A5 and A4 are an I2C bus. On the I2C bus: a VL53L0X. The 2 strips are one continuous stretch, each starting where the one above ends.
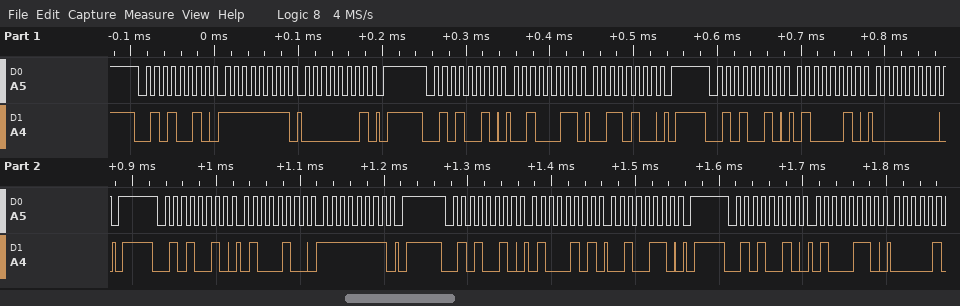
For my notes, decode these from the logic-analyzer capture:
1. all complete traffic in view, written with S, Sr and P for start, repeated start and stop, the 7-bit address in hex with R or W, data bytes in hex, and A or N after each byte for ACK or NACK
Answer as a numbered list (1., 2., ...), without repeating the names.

1. S 29W A FF A 01 A P S 29W A 23 A 34 A P S 29W A 42 A 00 A P S 29W A 44 A FF A P S 29W A 45 A 26 A P S 29W A 46 A
